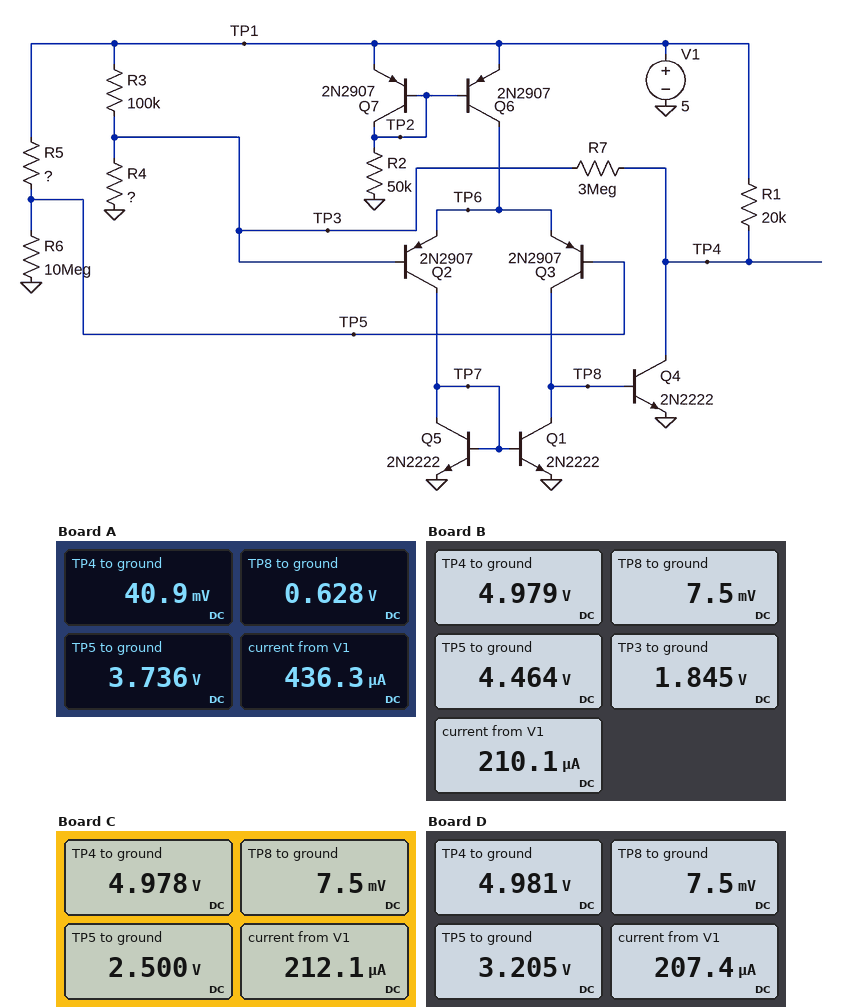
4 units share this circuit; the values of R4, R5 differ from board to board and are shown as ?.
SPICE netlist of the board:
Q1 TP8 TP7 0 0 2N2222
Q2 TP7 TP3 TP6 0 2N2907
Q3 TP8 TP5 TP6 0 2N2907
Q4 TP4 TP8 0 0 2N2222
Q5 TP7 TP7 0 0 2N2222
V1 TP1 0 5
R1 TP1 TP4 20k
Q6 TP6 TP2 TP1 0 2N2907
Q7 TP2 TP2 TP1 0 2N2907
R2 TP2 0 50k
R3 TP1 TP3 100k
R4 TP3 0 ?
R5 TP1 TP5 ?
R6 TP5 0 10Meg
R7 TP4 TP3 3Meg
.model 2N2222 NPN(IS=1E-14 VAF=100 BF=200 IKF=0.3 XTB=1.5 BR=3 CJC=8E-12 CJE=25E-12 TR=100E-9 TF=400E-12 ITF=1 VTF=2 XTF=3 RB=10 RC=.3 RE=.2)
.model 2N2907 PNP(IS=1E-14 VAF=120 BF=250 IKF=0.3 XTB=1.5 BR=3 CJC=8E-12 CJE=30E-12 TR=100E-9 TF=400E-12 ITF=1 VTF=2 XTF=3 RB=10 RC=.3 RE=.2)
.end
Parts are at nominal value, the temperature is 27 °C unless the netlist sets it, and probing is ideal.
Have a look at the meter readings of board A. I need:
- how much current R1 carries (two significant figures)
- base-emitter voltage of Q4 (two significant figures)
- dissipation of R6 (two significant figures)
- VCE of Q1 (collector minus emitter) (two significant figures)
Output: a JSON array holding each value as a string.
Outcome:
["250 µA", "630 mV", "1.4 µW", "630 mV"]
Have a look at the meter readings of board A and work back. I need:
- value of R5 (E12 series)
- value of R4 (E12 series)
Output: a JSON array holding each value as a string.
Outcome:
["8.2 MΩ", "330 kΩ"]
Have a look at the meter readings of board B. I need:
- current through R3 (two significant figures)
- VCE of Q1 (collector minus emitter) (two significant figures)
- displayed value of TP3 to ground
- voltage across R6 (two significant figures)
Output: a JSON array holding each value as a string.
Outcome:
["32 µA", "7.5 mV", "1.845 V", "4.5 V"]
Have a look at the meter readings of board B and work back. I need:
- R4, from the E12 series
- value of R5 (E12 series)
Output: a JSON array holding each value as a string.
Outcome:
["56 kΩ", "1.2 MΩ"]
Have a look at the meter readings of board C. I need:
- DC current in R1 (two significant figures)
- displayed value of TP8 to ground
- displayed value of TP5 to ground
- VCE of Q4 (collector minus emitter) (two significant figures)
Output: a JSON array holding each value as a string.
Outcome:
["1.1 µA", "7.5 mV", "2.500 V", "5.0 V"]
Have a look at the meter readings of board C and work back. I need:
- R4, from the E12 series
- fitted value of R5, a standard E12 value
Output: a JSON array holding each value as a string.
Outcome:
["47 kΩ", "10 MΩ"]
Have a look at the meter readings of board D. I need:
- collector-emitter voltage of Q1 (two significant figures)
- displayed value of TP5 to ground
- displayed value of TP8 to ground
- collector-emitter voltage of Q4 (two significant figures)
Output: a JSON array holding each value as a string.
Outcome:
["7.5 mV", "3.205 V", "7.5 mV", "5.0 V"]
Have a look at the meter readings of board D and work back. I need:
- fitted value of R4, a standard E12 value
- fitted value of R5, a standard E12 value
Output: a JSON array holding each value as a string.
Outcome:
["68 kΩ", "5.6 MΩ"]
